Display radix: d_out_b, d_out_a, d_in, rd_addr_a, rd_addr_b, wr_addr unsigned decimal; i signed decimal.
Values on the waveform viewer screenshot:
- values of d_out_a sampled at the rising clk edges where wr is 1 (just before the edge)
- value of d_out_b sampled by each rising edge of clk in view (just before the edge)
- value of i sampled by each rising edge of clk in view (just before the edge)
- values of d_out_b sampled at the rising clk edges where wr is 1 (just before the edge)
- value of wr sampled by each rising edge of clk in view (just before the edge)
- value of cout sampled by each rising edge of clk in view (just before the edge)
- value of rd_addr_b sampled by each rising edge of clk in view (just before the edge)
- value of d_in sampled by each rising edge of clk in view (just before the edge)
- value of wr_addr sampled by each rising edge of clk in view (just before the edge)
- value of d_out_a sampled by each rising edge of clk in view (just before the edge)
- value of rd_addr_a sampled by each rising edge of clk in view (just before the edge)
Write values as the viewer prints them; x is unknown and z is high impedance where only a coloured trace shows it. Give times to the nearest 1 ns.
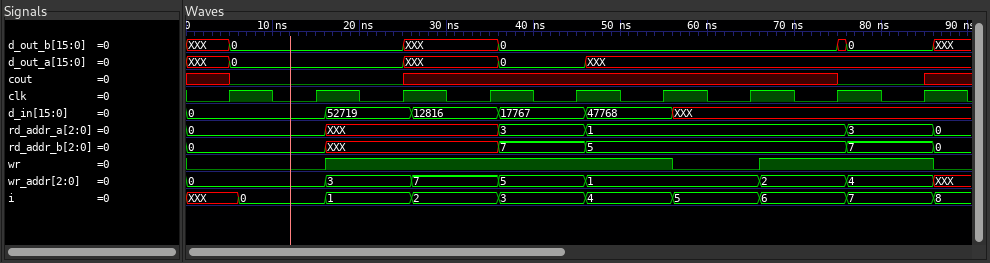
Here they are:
0, XXX, 0, XXX, XXX, XXX
XXX, 0, 0, XXX, 0, 0, 0, 0, 0
XXX, 0, 1, 2, 3, 4, 5, 6, 7
0, XXX, 0, 0, 0, 0
0 0 1 1 1 1 0 1 1
x 0 0 x x x x x 0
0, 0, XXX, XXX, 7, 5, 5, 5, 7
0, 0, 52719, 12816, 17767, 47768, XXX, XXX, XXX
0, 0, 3, 7, 5, 1, 1, 2, 4
XXX, 0, 0, XXX, 0, XXX, XXX, XXX, XXX
0, 0, XXX, XXX, 3, 1, 1, 1, 3
